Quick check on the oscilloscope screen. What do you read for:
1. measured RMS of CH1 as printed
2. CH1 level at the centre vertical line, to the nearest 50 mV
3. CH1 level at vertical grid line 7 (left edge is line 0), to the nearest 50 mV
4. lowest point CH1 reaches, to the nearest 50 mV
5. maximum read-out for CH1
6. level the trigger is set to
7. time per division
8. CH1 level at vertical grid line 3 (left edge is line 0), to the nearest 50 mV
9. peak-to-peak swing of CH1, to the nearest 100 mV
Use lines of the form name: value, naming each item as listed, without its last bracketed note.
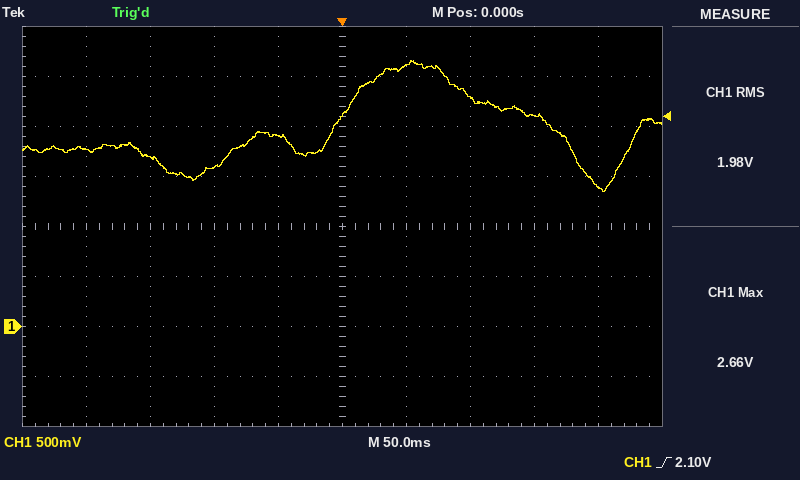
measured RMS of CH1 as printed: 1.98 V
CH1 level at the centre vertical line, to the nearest 50 mV: 2.10 V
CH1 level at vertical grid line 7 (left edge is line 0), to the nearest 50 mV: 2.30 V
lowest point CH1 reaches, to the nearest 50 mV: 1.35 V
maximum read-out for CH1: 2.66 V
level the trigger is set to: 2.10 V
time per division: 50 ms
CH1 level at vertical grid line 3 (left edge is line 0), to the nearest 50 mV: 1.60 V
peak-to-peak swing of CH1, to the nearest 100 mV: 1.30 V
